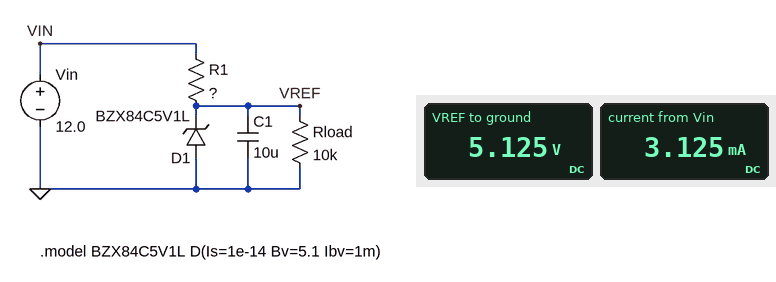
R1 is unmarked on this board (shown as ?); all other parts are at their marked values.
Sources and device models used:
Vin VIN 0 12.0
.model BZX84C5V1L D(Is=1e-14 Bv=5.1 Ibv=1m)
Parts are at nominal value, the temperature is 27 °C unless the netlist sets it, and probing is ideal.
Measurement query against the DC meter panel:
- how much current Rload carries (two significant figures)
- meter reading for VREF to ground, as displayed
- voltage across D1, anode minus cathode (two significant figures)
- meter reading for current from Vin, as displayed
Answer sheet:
510 µA
5.125 V
-5.1 V
3.125 mA
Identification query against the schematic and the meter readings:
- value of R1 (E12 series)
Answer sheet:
2.2 kΩ
